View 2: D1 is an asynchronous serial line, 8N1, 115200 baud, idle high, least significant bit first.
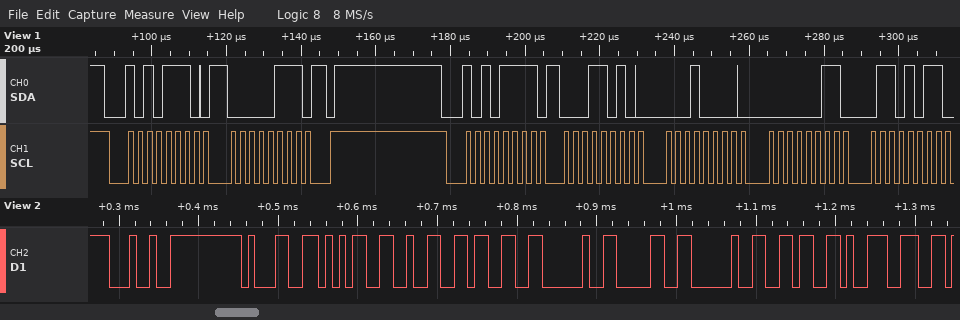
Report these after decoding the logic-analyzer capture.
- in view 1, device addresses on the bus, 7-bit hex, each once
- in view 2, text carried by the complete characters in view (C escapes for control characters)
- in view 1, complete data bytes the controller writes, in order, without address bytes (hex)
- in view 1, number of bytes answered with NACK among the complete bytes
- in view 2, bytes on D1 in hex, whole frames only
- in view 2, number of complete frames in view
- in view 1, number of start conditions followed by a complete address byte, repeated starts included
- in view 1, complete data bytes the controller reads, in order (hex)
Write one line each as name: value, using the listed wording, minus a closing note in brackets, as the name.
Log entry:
in view 1, device addresses on the bus, 7-bit hex, each once: 0x57
in view 2, text carried by the complete characters in view: "$1523 0 69"
in view 1, complete data bytes the controller writes, in order, without address bytes: 07
in view 1, number of bytes answered with NACK among the complete bytes: 0
in view 2, bytes on D1 in hex, whole frames only: 24 31 35 32 33 20 30 20 36 39
in view 2, number of complete frames in view: 10
in view 1, number of start conditions followed by a complete address byte, repeated starts included: 2
in view 1, complete data bytes the controller reads, in order: 1A 10 03 6B
